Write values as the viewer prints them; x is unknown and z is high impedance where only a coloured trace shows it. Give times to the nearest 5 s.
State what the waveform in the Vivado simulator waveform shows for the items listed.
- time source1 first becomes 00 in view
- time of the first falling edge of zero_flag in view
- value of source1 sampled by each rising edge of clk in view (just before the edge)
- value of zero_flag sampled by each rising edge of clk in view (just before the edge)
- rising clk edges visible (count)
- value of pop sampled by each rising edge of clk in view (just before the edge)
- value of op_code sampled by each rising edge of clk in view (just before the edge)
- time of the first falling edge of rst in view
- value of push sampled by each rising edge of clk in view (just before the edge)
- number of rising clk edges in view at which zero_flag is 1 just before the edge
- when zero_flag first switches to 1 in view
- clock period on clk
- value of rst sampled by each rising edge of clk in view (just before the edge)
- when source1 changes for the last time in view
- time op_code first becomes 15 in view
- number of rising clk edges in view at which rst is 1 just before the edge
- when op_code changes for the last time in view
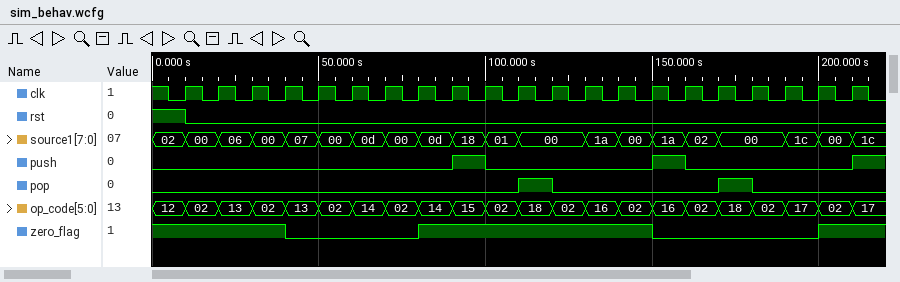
10 s
40 s
02, 00, 06, 00, 07, 00, 0d, 00, 0d, 18, 01, 00, 00, 1a, 00, 1a, 02, 00, 00, 1c, 00
1 1 1 1 0 0 0 0 1 1 1 1 1 1 1 0 0 0 0 0 1
21
0 0 0 0 0 0 0 0 0 0 0 1 0 0 0 0 0 1 0 0 0
12, 02, 13, 02, 13, 02, 14, 02, 14, 15, 02, 18, 02, 16, 02, 16, 02, 18, 02, 17, 02
10 s
0 0 0 0 0 0 0 0 0 1 0 0 0 0 0 1 0 0 0 0 0
12
80 s
10 s
1 0 0 0 0 0 0 0 0 0 0 0 0 0 0 0 0 0 0 0 0
210 s
90 s
1
210 s
